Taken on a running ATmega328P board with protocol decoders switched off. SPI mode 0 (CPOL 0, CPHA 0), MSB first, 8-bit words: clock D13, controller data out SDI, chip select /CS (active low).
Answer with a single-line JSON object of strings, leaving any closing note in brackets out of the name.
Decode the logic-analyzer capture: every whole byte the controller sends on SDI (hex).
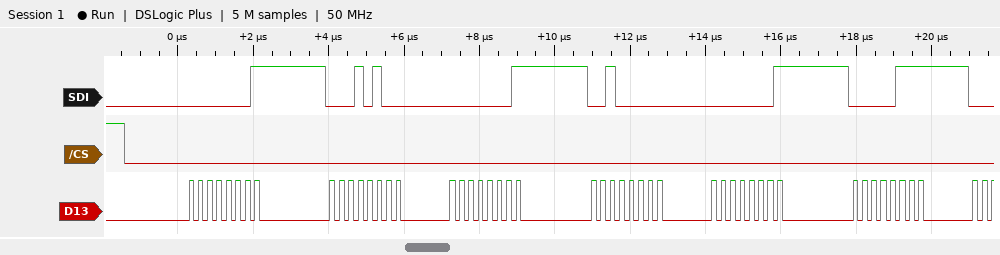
{"every whole byte the controller sends on SDI": "01 14 01 20 01 07"}
